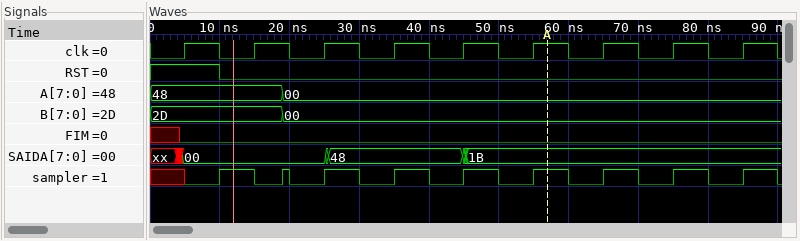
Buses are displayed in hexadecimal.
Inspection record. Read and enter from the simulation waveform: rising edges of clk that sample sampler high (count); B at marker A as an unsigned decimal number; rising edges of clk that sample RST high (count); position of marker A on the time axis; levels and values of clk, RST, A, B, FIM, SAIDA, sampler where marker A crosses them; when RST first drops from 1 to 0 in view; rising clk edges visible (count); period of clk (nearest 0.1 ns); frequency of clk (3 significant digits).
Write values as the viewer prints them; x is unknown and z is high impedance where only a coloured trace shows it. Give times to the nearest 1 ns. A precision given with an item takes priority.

1
0
1
57 ns
clk=1, RST=0, A=00, B=00, FIM=0, SAIDA=1B, sampler=1
10 ns
9
10 ns
100 MHz
